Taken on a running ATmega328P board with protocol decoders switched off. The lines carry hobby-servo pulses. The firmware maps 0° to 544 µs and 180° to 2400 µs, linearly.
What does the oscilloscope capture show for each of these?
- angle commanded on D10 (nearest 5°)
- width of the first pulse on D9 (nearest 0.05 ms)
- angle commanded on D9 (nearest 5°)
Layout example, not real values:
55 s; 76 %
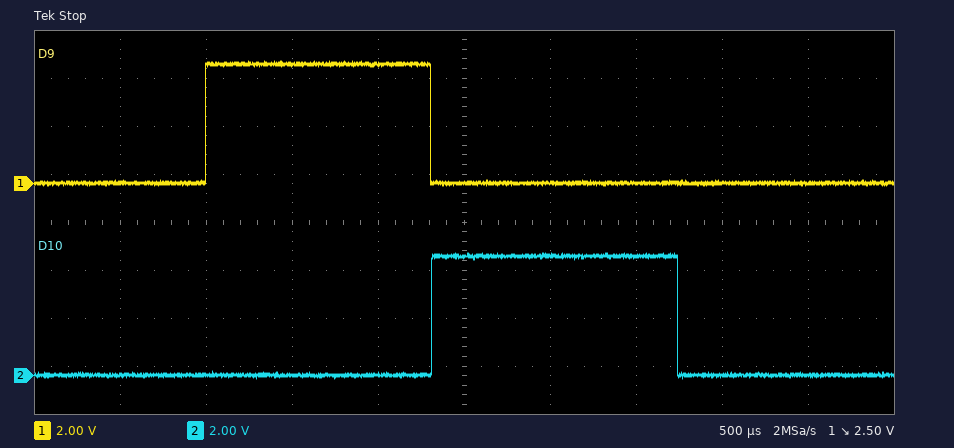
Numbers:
85°; 1.30 ms; 75°
